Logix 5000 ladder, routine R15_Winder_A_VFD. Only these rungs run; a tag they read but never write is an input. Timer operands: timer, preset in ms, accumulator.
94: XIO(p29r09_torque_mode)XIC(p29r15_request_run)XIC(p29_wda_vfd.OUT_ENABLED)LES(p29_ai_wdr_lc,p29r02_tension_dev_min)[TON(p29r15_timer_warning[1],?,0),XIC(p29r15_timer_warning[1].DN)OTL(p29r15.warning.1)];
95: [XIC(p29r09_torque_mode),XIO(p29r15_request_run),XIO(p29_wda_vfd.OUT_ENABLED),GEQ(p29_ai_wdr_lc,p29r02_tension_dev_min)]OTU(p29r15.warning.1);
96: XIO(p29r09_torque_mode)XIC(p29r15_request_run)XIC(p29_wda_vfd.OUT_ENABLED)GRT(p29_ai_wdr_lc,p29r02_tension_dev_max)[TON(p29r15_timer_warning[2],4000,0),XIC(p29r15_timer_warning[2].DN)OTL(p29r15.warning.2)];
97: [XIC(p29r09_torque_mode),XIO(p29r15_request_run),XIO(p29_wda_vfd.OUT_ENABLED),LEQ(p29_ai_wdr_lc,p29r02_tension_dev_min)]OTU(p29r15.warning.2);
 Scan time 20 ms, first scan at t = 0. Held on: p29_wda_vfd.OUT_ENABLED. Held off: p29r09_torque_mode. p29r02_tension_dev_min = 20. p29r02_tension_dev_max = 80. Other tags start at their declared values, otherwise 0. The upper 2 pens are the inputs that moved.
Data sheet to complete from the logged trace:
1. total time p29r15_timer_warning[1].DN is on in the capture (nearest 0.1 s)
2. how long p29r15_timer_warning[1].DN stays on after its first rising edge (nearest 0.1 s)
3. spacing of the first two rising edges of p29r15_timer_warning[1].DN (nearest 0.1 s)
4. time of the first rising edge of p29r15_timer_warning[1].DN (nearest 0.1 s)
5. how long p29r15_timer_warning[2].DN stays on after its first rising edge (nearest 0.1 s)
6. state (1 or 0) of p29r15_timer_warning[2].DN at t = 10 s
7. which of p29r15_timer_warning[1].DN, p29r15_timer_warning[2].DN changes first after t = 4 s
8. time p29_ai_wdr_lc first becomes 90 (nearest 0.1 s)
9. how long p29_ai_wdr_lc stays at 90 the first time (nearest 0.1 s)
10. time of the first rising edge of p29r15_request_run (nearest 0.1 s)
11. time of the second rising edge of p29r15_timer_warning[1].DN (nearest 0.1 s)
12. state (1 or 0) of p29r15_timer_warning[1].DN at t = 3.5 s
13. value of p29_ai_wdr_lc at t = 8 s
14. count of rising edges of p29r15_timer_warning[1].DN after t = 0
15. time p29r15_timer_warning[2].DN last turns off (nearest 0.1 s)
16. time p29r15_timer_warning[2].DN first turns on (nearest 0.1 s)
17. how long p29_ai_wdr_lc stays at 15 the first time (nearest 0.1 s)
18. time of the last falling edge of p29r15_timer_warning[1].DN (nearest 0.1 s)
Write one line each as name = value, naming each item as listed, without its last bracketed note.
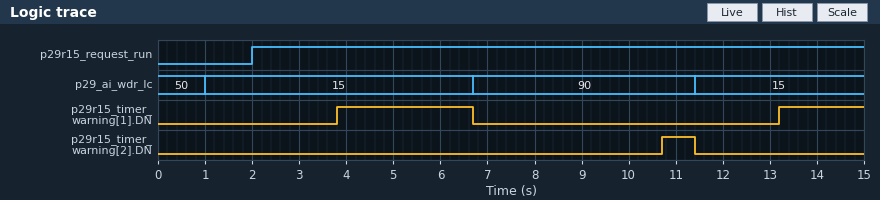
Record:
total time p29r15_timer_warning[1].DN is on in the capture = 4.7 s
how long p29r15_timer_warning[1].DN stays on after its first rising edge = 2.9 s
spacing of the first two rising edges of p29r15_timer_warning[1].DN = 9.4 s
time of the first rising edge of p29r15_timer_warning[1].DN = 3.8 s
how long p29r15_timer_warning[2].DN stays on after its first rising edge = 0.7 s
state (1 or 0) of p29r15_timer_warning[2].DN at t = 10 s = 0
which of p29r15_timer_warning[1].DN, p29r15_timer_warning[2].DN changes first after t = 4 s = p29r15_timer_warning[1].DN
time p29_ai_wdr_lc first becomes 90 = 6.7 s
how long p29_ai_wdr_lc stays at 90 the first time = 4.7 s
time of the first rising edge of p29r15_request_run = 2.0 s
time of the second rising edge of p29r15_timer_warning[1].DN = 13.2 s
state (1 or 0) of p29r15_timer_warning[1].DN at t = 3.5 s = 0
value of p29_ai_wdr_lc at t = 8 s = 90
count of rising edges of p29r15_timer_warning[1].DN after t = 0 = 2
time p29r15_timer_warning[2].DN last turns off = 11.4 s
time p29r15_timer_warning[2].DN first turns on = 10.7 s
how long p29_ai_wdr_lc stays at 15 the first time = 5.7 s
time of the last falling edge of p29r15_timer_warning[1].DN = 6.7 s
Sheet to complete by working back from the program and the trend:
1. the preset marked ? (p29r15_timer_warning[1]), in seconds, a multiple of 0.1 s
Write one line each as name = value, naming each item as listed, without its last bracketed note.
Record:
the preset marked ? (p29r15_timer_warning[1]), in seconds, a multiple of 0.1 s = 1.8 s
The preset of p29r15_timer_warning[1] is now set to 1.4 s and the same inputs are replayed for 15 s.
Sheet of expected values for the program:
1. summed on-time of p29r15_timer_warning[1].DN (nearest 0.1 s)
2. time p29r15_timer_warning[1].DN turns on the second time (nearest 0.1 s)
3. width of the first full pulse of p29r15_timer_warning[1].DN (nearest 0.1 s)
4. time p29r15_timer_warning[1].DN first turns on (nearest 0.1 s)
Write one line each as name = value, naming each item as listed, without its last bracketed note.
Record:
summed on-time of p29r15_timer_warning[1].DN = 5.5 s
time p29r15_timer_warning[1].DN turns on the second time = 12.8 s
width of the first full pulse of p29r15_timer_warning[1].DN = 3.3 s
time p29r15_timer_warning[1].DN first turns on = 3.4 s
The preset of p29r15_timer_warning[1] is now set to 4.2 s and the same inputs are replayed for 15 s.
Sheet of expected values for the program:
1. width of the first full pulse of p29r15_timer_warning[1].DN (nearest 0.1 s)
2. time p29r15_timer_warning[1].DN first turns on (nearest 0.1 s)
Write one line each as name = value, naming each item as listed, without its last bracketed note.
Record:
width of the first full pulse of p29r15_timer_warning[1].DN = 0.5 s
time p29r15_timer_warning[1].DN first turns on = 6.2 s
